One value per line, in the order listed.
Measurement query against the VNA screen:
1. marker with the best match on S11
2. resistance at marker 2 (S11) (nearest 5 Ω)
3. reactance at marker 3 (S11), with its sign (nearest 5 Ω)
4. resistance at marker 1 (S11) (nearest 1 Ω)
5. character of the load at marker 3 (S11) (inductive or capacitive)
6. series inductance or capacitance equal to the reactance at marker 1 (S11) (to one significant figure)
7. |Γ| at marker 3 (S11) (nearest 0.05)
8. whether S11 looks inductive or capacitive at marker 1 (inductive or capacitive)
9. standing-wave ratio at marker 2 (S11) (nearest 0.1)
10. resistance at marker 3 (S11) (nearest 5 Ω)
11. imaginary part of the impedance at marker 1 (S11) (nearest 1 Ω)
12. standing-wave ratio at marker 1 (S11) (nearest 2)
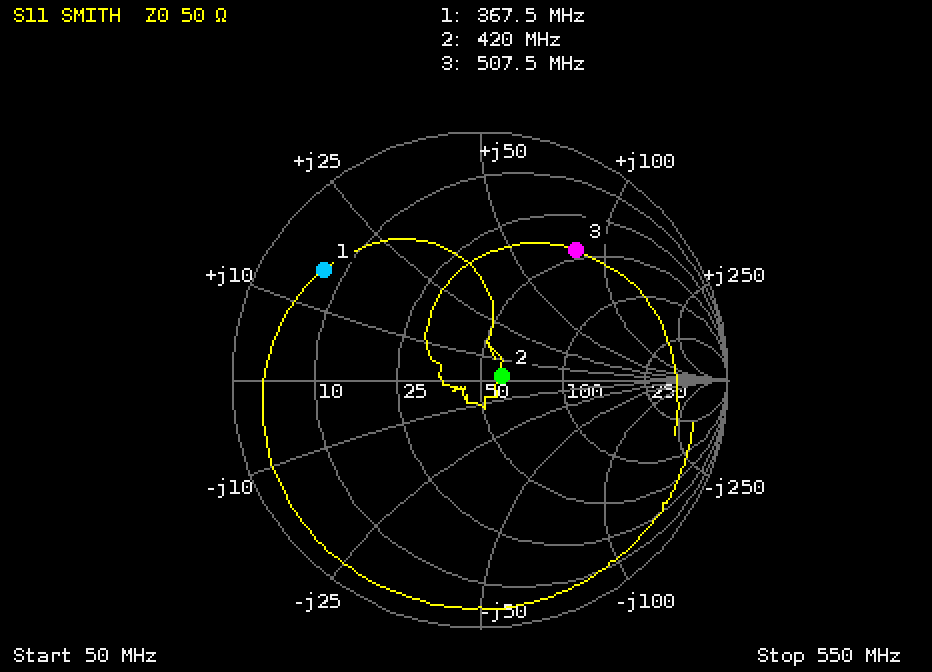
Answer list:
marker 2
60 Ω
+80 Ω
7 Ω
inductive
7 nH
0.65
inductive
1.2
45 Ω
+16 Ω
8
